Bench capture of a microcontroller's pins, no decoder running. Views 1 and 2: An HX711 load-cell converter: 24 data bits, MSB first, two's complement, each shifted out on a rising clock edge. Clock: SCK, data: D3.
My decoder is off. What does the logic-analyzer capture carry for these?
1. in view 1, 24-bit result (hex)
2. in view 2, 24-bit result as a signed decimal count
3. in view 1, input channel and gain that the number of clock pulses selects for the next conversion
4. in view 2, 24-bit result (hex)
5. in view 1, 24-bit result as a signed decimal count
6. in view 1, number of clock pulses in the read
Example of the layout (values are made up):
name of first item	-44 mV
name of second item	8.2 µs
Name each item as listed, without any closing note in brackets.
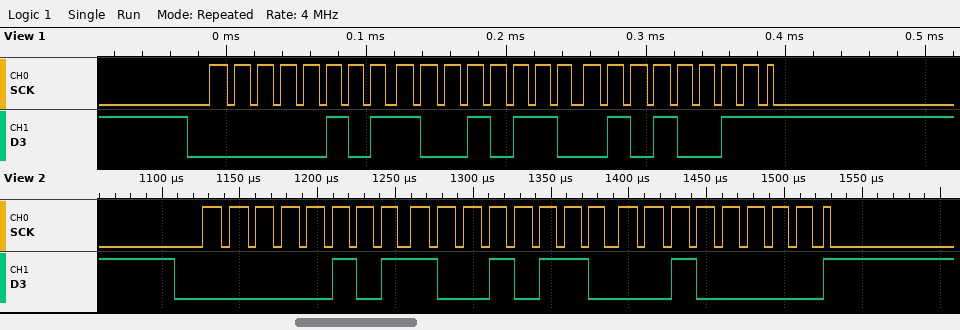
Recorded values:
in view 1, 24-bit result	0x059653
in view 2, 24-bit result as a signed decimal count	366112
in view 1, input channel and gain that the number of clock pulses selects for the next conversion	channel A, gain 128
in view 2, 24-bit result	0x059620
in view 1, 24-bit result as a signed decimal count	366163
in view 1, number of clock pulses in the read	25
